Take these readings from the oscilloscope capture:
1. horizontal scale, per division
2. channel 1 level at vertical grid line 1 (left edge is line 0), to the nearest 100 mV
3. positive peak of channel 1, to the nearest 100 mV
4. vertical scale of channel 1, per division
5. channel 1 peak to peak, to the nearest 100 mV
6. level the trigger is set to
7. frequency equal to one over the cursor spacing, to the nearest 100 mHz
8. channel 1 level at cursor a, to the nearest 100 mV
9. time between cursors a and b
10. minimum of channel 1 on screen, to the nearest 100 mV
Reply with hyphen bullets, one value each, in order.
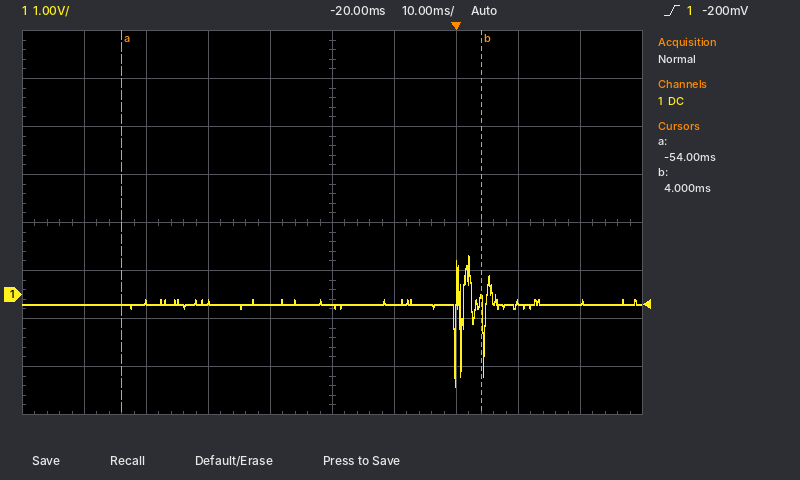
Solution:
- 10 ms
- -200 mV
- 800 mV
- 1 V
- 2.7 V
- -200 mV
- 17.2 Hz
- -200 mV
- 58 ms
- -1.9 V
